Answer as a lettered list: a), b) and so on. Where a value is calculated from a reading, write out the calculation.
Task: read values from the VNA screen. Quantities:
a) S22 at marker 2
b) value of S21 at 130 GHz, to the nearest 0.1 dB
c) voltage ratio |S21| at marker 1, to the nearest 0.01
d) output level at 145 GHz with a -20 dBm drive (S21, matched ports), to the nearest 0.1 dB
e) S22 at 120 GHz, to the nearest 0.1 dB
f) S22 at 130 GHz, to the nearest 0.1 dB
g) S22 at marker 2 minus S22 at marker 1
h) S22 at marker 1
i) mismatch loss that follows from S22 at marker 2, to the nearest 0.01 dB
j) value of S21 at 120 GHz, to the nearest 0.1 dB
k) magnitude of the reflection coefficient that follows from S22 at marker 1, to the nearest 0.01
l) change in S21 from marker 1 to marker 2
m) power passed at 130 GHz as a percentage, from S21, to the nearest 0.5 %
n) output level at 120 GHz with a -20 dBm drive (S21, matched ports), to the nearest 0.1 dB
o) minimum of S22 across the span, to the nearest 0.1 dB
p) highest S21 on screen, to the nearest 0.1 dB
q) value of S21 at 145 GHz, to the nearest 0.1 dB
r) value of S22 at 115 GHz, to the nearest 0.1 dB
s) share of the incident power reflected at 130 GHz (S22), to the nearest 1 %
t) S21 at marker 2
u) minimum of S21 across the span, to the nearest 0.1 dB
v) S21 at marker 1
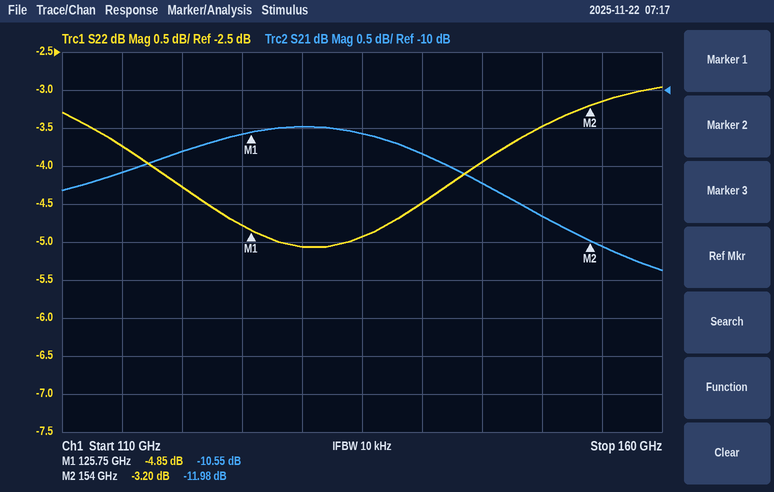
a) -3.20 dB
b) -10.5 dB
c) 10^(-10.55/20) ≈ 0.30
d) -20 dBm + (-11.2 dB) = -31.2 dBm
e) -4.3 dB
f) -5.1 dB
g) -3.2 − (-4.85) = 1.65 dB
h) -4.85 dB
i) −10 log10(1 − 10^(-3.2/10)) ≈ 2.83 dB
j) -10.8 dB
k) 10^(-4.85/20) ≈ 0.57
l) -11.98 − (-10.55) = -1.43 dB
m) 10^(-10.5/10) ≈ 8.91 %, so 9.0 % to the nearest 0.5 %
n) -20 dBm + (-10.8 dB) = -30.8 dBm
o) -5.1 dB
p) -10.5 dB
q) -11.2 dB
r) -3.7 dB
s) 10^(-5.1/10) ≈ 31 %
t) -11.98 dB
u) -12.4 dB
v) -10.55 dB
